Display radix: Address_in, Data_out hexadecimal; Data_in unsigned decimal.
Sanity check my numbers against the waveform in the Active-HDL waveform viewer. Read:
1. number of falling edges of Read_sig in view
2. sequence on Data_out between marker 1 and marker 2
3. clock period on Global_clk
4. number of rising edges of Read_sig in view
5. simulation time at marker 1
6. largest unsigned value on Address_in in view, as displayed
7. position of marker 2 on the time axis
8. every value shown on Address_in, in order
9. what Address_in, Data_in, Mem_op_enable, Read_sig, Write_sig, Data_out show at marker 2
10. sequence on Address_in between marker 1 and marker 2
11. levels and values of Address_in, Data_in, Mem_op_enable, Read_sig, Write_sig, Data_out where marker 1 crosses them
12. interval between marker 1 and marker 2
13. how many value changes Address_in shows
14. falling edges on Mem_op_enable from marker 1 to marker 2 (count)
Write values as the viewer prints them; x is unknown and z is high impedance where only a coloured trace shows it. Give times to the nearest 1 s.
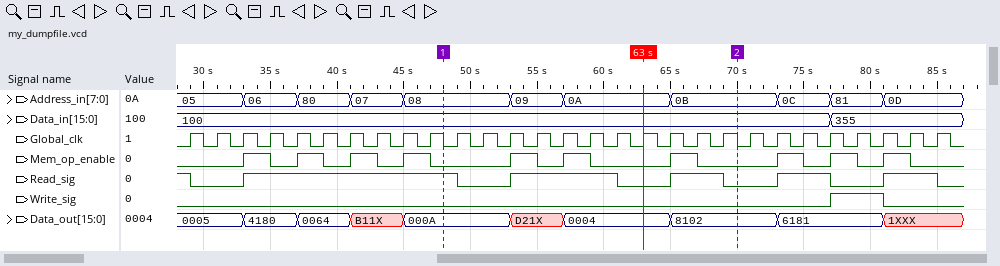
6
000A, D21X, 0004, 8102
2 s
5
48 s
81
70 s
05, 06, 80, 07, 08, 09, 0A, 0B, 0C, 81, 0D
Address_in=0B, Data_in=100, Mem_op_enable=0, Read_sig=0, Write_sig=0, Data_out=8102
08, 09, 0A, 0B
Address_in=08, Data_in=100, Mem_op_enable=0, Read_sig=1, Write_sig=0, Data_out=000A
22 s
10
3
